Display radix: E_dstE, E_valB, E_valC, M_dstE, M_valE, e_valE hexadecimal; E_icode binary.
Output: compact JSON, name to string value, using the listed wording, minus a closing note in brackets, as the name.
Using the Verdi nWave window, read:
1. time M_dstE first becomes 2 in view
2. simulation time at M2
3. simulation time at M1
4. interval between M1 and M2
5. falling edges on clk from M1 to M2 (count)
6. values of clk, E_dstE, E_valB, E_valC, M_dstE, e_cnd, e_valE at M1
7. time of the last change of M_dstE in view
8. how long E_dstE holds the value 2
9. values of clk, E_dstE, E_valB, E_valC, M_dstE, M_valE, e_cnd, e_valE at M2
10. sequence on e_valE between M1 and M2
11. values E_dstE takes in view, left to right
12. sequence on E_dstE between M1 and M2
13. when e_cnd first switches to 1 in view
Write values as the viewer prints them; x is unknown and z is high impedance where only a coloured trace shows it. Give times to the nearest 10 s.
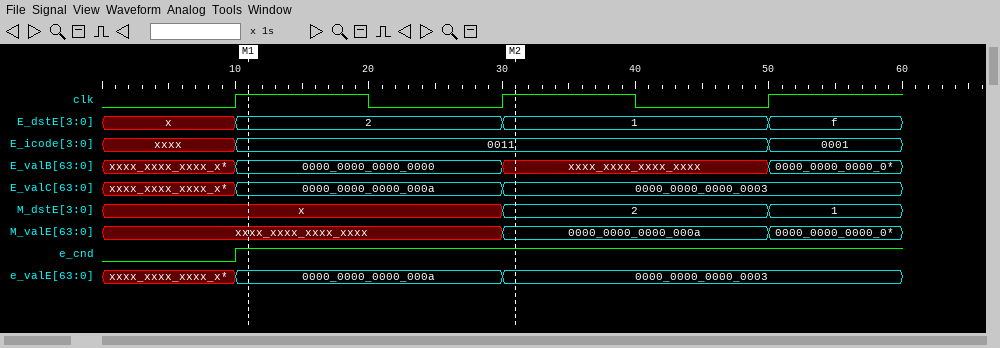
{"time M_dstE first becomes 2 in view": "30 s", "simulation time at M2": "30 s", "simulation time at M1": "10 s", "interval between M1 and M2": "20 s", "falling edges on clk from M1 to M2": "1", "values of clk, E_dstE, E_valB, E_valC, M_dstE, e_cnd, e_valE at M1": "clk=1, E_dstE=2, E_valB=0000_0000_0000_0000, E_valC=0000_0000_0000_000a, M_dstE=x, e_cnd=1, e_valE=0000_0000_0000_000a", "time of the last change of M_dstE in view": "50 s", "how long E_dstE holds the value 2": "20 s", "values of clk, E_dstE, E_valB, E_valC, M_dstE, M_valE, e_cnd, e_valE at M2": "clk=1, E_dstE=1, E_valB=xxxx_xxxx_xxxx_xxxx, E_valC=0000_0000_0000_0003, M_dstE=2, M_valE=0000_0000_0000_000a, e_cnd=1, e_valE=0000_0000_0000_0003", "sequence on e_valE between M1 and M2": "0000_0000_0000_000a, 0000_0000_0000_0003", "values E_dstE takes in view, left to right": "x, 2, 1, f", "sequence on E_dstE between M1 and M2": "2, 1", "when e_cnd first switches to 1 in view": "10 s"}
